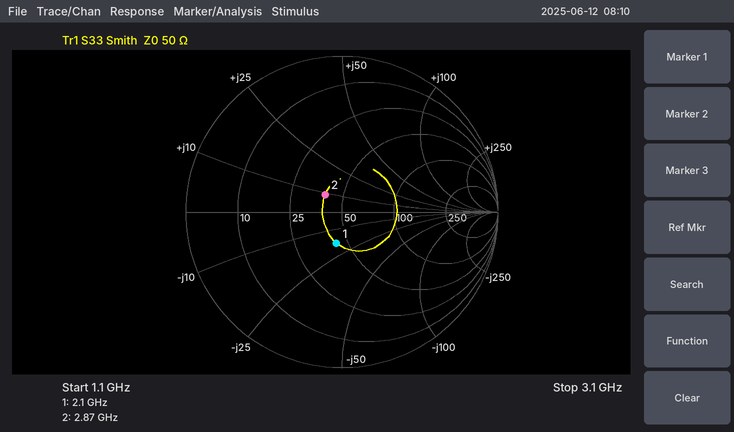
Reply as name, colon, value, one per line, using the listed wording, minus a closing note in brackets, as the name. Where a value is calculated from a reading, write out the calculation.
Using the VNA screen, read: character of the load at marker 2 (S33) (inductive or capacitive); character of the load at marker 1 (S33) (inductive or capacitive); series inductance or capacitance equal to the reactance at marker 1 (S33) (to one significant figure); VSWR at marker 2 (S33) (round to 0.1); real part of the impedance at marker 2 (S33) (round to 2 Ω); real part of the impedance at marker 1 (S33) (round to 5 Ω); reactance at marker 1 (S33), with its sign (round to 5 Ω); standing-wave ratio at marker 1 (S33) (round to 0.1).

character of the load at marker 2 (S33): inductive
character of the load at marker 1 (S33): capacitive
series inductance or capacitance equal to the reactance at marker 1 (S33): C = 1/(2π × 2.1 GHz × 20 Ω) ≈ 4 pF
VSWR at marker 2 (S33): 1.4
real part of the impedance at marker 2 (S33): 40 Ω
real part of the impedance at marker 1 (S33): 45 Ω
reactance at marker 1 (S33), with its sign: -20 Ω
standing-wave ratio at marker 1 (S33): 1.5
